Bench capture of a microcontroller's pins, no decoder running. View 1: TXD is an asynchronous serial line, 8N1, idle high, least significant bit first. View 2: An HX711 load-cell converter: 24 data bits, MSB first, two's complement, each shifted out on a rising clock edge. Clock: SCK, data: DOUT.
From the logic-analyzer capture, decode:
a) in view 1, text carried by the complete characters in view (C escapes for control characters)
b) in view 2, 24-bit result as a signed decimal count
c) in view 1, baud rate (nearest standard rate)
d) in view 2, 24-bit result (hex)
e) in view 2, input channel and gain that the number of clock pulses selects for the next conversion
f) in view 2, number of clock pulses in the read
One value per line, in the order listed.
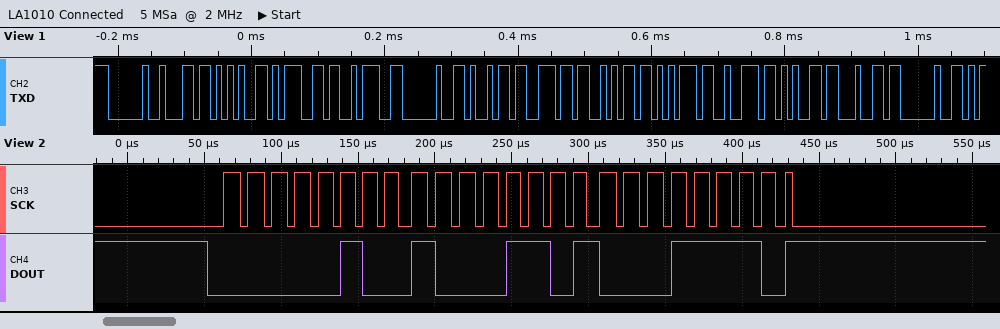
" leg: injured "
298270
115200 baud
0x048D1E
channel A, gain 128
25
